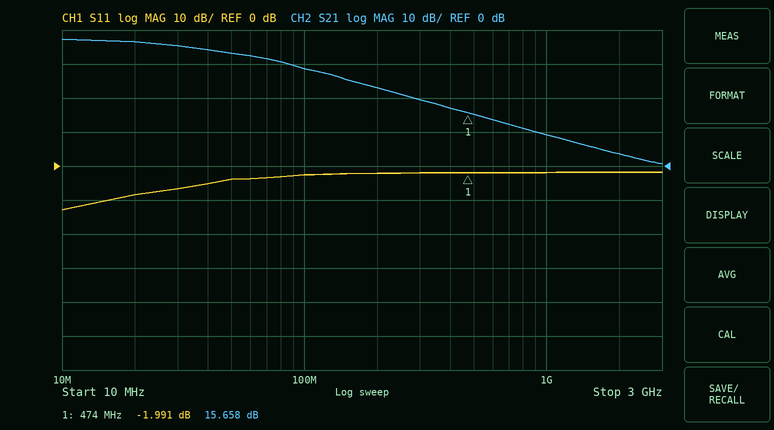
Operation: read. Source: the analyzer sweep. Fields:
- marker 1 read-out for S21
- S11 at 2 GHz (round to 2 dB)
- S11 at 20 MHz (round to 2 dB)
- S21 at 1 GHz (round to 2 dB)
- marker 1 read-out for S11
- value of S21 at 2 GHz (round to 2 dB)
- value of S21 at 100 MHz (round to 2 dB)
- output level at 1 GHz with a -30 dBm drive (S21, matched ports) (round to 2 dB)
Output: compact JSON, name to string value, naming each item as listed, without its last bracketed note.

{"marker 1 read-out for S21": "15.658 dB", "S11 at 2 GHz": "-2 dB", "S11 at 20 MHz": "-8 dB", "S21 at 1 GHz": "10 dB", "marker 1 read-out for S11": "-1.991 dB", "value of S21 at 2 GHz": "4 dB", "value of S21 at 100 MHz": "28 dB", "output level at 1 GHz with a -30 dBm drive (S21, matched ports)": "-20 dBm"}
